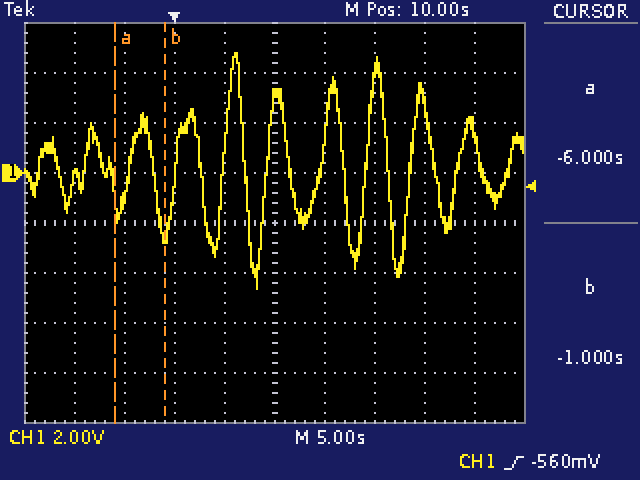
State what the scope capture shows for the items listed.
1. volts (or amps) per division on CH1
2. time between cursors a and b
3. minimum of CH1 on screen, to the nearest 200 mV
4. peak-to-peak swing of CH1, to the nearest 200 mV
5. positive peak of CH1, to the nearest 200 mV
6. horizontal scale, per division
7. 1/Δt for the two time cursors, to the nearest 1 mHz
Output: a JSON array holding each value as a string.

["2 V", "5.0 s", "-4.6 V", "9.4 V", "4.8 V", "5 s", "200 mHz"]
